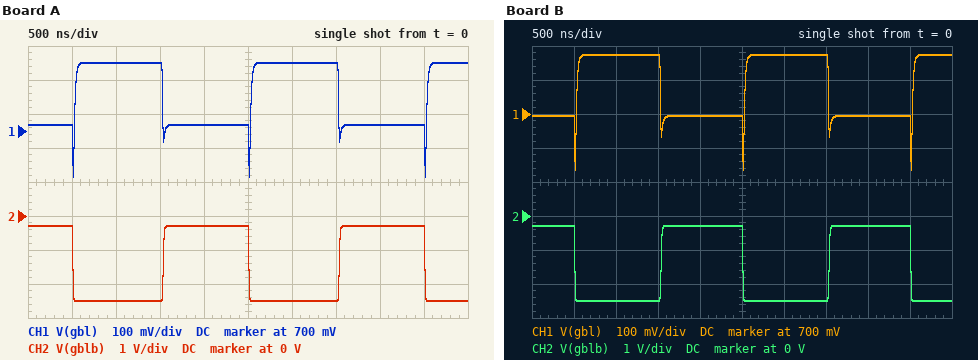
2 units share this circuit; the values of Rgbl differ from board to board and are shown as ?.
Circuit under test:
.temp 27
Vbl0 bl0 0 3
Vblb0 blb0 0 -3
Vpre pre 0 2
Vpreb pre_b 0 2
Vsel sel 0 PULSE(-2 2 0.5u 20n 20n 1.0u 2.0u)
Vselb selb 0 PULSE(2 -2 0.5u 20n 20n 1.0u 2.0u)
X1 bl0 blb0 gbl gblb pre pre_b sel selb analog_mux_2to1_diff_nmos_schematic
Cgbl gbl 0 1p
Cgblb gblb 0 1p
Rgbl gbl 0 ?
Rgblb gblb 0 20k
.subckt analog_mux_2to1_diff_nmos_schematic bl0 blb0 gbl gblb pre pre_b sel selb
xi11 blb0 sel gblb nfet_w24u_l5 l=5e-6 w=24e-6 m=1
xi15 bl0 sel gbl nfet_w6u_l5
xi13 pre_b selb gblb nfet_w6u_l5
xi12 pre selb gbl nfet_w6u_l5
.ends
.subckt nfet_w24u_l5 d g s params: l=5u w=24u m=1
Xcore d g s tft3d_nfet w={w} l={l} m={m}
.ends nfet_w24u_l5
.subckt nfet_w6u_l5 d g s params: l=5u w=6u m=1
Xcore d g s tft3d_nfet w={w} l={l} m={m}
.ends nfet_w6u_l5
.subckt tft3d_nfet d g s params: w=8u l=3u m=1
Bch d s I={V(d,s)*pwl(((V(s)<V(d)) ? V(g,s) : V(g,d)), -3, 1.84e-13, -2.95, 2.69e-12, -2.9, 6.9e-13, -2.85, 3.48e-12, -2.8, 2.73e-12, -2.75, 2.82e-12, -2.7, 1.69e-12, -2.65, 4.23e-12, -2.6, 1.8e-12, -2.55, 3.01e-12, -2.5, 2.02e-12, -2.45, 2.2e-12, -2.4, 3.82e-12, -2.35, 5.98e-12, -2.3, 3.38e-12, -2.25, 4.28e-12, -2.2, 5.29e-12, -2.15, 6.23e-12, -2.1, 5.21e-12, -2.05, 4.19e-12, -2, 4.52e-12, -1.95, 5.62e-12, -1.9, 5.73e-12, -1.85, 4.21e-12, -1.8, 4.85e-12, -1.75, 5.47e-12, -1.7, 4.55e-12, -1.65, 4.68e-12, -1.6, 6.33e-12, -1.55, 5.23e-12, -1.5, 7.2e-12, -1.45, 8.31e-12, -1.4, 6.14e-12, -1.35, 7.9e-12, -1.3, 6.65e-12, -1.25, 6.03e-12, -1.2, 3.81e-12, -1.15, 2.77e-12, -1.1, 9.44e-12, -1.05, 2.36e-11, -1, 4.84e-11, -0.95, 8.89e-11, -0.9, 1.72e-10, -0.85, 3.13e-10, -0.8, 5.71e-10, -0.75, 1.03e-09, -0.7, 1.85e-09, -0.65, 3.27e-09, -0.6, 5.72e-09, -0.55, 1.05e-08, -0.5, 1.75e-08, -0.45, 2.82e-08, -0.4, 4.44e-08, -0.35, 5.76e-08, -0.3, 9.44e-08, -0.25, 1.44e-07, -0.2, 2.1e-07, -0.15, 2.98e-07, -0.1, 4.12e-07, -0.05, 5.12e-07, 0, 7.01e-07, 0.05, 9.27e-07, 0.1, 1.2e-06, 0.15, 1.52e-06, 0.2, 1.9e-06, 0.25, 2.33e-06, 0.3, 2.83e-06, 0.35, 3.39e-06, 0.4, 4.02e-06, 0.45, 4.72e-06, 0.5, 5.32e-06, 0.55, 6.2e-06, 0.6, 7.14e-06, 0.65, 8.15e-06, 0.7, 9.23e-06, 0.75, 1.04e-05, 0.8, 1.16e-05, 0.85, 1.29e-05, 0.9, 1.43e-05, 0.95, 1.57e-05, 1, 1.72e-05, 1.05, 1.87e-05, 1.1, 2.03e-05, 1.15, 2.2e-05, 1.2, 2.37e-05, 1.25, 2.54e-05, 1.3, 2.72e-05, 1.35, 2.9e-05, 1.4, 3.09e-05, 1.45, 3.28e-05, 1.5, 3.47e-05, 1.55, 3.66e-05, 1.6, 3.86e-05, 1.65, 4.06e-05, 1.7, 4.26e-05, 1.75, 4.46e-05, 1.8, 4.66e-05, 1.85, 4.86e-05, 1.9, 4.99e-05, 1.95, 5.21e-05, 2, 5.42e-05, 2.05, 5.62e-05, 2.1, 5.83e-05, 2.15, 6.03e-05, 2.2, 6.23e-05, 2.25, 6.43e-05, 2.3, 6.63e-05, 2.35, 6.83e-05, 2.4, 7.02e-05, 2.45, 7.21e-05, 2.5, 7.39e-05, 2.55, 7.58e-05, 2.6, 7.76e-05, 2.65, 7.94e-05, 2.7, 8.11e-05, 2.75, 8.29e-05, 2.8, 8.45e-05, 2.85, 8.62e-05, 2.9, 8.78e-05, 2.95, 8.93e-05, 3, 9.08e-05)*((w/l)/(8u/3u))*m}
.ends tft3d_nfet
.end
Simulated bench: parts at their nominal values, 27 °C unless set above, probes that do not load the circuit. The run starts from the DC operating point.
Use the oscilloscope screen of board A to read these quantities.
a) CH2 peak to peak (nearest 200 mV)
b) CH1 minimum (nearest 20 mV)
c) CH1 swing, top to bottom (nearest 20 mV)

2.2 V
560 mV
340 mV
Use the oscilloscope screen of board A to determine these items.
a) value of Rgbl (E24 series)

47 kΩ
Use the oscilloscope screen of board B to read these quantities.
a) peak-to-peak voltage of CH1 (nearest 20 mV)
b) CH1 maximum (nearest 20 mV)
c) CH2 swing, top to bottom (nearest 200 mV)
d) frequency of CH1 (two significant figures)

340 mV
880 mV
2.2 V
500 kHz
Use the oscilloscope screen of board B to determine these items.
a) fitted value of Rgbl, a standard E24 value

43 kΩ
